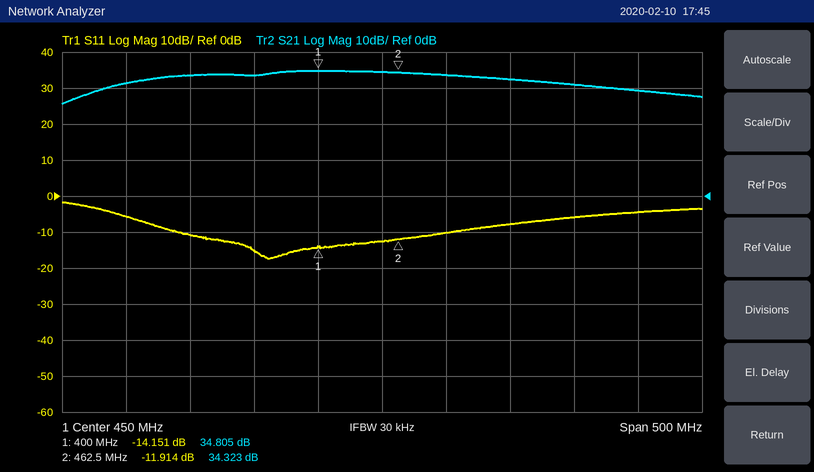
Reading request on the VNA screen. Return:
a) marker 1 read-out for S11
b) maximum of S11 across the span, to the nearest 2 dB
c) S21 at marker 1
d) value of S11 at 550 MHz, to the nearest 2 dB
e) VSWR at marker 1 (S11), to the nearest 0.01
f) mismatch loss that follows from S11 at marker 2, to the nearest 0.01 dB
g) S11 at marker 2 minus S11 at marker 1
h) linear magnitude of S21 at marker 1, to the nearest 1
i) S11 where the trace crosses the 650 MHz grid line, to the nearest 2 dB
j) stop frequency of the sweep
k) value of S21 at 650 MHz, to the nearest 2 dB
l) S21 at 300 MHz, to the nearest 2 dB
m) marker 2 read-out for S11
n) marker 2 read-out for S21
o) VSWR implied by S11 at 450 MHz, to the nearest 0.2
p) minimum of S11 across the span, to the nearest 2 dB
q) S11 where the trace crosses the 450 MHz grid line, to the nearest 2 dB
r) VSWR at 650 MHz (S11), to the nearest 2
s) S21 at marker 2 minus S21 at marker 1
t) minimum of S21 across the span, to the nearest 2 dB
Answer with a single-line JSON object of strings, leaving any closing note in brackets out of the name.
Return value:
{"marker 1 read-out for S11": "-14.151 dB", "maximum of S11 across the span, to the nearest 2 dB": "-2 dB", "S21 at marker 1": "34.805 dB", "value of S11 at 550 MHz, to the nearest 2 dB": "-8 dB", "VSWR at marker 1 (S11), to the nearest 0.01": "1.49", "mismatch loss that follows from S11 at marker 2, to the nearest 0.01 dB": "0.29 dB", "S11 at marker 2 minus S11 at marker 1": "2.237 dB", "linear magnitude of S21 at marker 1, to the nearest 1": "55", "S11 where the trace crosses the 650 MHz grid line, to the nearest 2 dB": "-4 dB", "stop frequency of the sweep": "700 MHz", "value of S21 at 650 MHz, to the nearest 2 dB": "30 dB", "S21 at 300 MHz, to the nearest 2 dB": "34 dB", "marker 2 read-out for S11": "-11.914 dB", "marker 2 read-out for S21": "34.323 dB", "VSWR implied by S11 at 450 MHz, to the nearest 0.2": "1.6", "minimum of S11 across the span, to the nearest 2 dB": "-18 dB", "S11 where the trace crosses the 450 MHz grid line, to the nearest 2 dB": "-12 dB", "VSWR at 650 MHz (S11), to the nearest 2": "4", "S21 at marker 2 minus S21 at marker 1": "-0.482 dB", "minimum of S21 across the span, to the nearest 2 dB": "26 dB"}
